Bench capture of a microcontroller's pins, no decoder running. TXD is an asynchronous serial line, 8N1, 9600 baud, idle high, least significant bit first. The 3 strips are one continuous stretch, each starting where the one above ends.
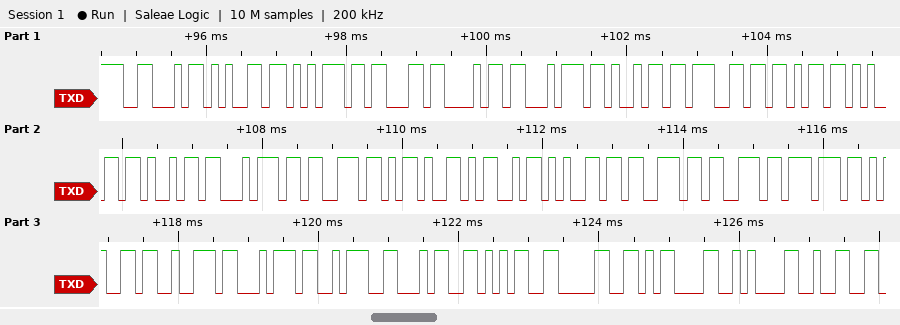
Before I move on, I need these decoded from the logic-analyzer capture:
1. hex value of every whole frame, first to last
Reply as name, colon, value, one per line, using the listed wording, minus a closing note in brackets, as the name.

hex value of every whole frame, first to last: 46 65 75 63 68 74 69 67 6B 65 69 74 73 2D 4D 65 73 73 77 65 72 74 3A 34 35 30 0D 0A 32
